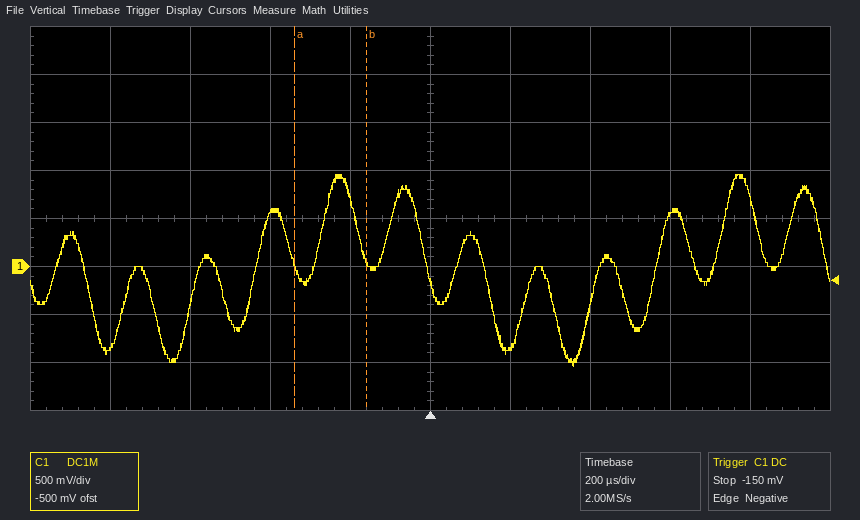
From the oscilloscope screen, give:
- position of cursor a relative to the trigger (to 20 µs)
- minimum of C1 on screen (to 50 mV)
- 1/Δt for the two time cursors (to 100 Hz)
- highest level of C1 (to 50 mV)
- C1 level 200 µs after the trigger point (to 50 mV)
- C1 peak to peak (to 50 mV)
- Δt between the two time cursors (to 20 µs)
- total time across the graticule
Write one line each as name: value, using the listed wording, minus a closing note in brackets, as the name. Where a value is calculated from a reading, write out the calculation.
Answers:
position of cursor a relative to the trigger: -340 µs
minimum of C1 on screen: -1.05 V
1/Δt for the two time cursors: 1 / 180 µs ≈ 5.6 kHz
highest level of C1: 950 mV
C1 level 200 µs after the trigger point: -850 mV
C1 peak to peak: 950 mV − (-1.05 V) = 2.00 V
Δt between the two time cursors: 180 µs
total time across the graticule: 2 ms
